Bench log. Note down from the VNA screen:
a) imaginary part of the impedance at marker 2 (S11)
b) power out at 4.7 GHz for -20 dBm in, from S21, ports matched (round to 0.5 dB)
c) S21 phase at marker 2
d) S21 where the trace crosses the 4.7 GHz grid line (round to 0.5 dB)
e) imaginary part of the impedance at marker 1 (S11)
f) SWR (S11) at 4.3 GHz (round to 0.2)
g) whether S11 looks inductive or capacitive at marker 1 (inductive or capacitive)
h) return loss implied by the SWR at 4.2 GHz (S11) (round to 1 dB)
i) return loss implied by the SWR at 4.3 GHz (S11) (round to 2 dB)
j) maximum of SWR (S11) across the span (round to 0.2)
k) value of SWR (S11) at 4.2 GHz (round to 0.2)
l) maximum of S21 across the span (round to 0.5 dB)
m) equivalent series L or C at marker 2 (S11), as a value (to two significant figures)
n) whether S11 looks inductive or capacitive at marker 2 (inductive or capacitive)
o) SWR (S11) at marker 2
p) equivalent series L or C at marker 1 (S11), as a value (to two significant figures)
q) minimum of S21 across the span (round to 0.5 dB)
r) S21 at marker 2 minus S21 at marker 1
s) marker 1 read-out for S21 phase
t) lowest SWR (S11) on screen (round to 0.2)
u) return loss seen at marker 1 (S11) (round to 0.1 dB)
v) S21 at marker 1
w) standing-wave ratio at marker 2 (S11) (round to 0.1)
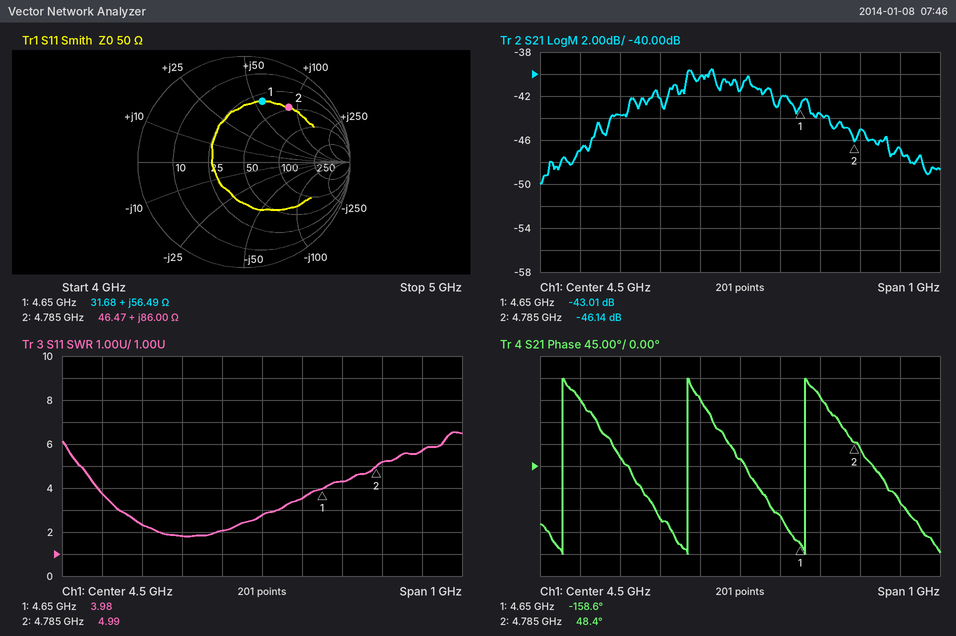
+86.00 Ω
-63.5 dBm
48.4°
-43.5 dB
+56.49 Ω
1.8
inductive
8 dB
10 dB
6.6
2.4
-39.5 dB
2.9 nH
inductive
4.99
1.9 nH
-50.0 dB
-3.13 dB
-158.6°
1.8
4.5 dB
-43.01 dB
5.0
